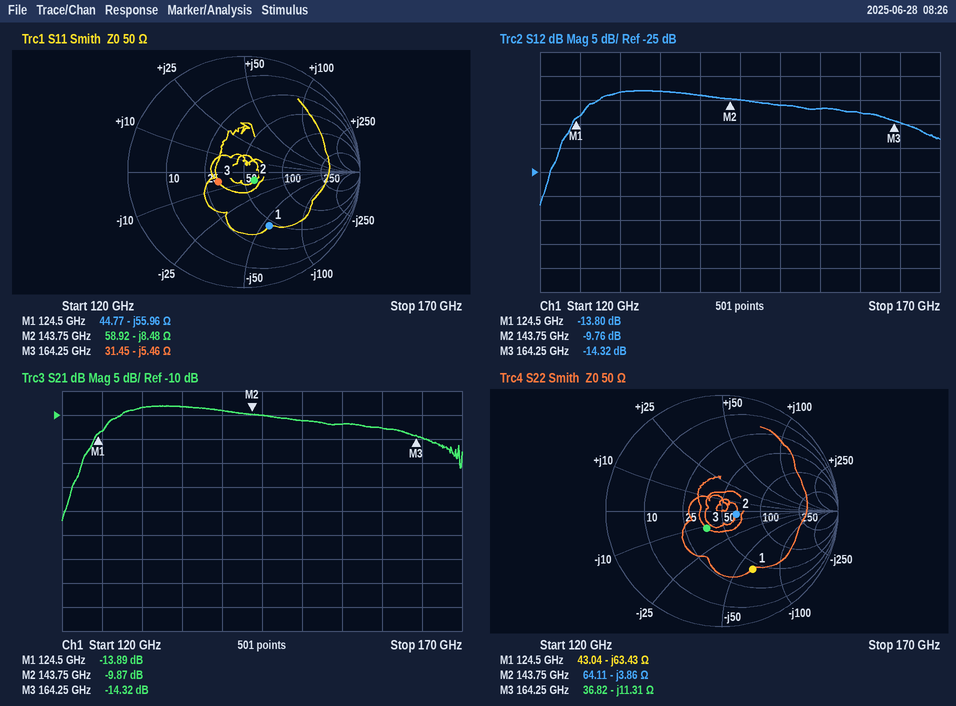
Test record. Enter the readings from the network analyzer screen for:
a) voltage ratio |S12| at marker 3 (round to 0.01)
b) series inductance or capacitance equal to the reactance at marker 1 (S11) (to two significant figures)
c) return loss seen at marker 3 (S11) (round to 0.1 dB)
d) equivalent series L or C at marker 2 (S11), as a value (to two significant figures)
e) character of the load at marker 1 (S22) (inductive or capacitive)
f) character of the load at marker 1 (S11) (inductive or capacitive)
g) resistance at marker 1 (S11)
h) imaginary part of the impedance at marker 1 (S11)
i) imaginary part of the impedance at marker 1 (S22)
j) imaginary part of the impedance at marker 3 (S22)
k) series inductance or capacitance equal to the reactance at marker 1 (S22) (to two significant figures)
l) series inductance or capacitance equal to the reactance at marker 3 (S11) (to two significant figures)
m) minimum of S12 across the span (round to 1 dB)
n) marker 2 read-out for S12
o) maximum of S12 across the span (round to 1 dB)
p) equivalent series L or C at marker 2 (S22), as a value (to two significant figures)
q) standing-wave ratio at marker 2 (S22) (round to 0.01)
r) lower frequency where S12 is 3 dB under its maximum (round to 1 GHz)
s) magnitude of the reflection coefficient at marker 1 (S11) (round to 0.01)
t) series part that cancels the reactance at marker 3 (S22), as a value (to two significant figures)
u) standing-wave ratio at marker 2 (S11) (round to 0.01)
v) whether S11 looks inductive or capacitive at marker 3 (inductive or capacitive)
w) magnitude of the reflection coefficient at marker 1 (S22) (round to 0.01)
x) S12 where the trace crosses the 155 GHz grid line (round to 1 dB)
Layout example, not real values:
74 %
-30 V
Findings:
0.19
23 fF
12.5 dB
130 fF
capacitive
capacitive
44.77 Ω
-55.96 Ω
-63.43 Ω
-11.31 Ω
20 fF
180 fF
-32 dB
-9.76 dB
-8 dB
290 fF
1.29
126 GHz
0.51
11 pH
1.25
capacitive
0.57
-12 dB
